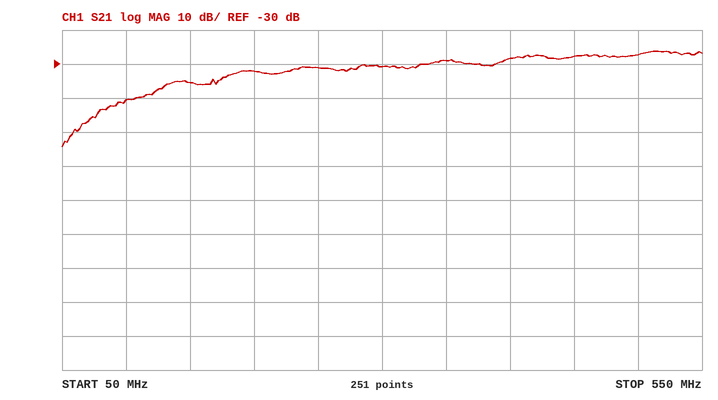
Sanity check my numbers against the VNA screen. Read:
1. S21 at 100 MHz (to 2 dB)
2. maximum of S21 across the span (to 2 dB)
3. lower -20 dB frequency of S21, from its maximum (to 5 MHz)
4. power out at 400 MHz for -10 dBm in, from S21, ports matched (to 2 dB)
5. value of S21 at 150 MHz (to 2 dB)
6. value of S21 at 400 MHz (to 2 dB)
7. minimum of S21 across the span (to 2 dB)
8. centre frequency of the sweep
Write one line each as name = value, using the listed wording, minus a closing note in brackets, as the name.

S21 at 100 MHz = -40 dB
maximum of S21 across the span = -26 dB
lower -20 dB frequency of S21, from its maximum = 70 MHz
power out at 400 MHz for -10 dBm in, from S21, ports matched = -38 dBm
value of S21 at 150 MHz = -36 dB
value of S21 at 400 MHz = -28 dB
minimum of S21 across the span = -54 dB
centre frequency of the sweep = 300 MHz
